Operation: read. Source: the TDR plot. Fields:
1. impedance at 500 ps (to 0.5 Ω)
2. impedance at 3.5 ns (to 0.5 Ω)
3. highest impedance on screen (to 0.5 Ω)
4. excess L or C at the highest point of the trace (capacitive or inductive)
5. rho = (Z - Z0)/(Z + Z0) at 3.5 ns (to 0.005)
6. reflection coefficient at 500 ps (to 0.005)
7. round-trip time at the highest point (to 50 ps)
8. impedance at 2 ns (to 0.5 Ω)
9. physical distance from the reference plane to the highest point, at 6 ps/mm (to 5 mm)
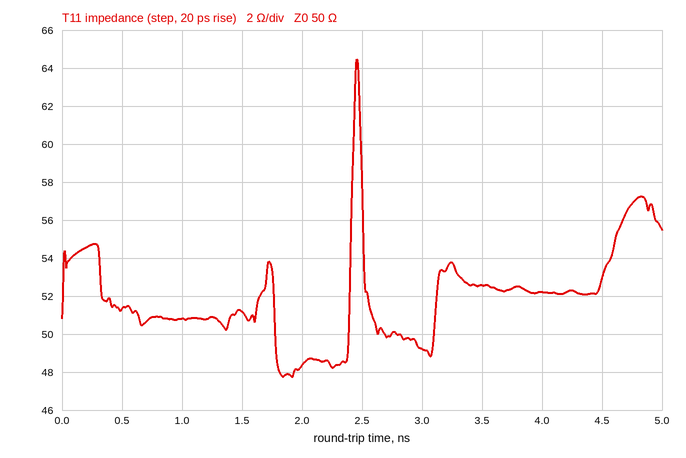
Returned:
51.5 Ω
52.5 Ω
64.5 Ω
inductive
+0.025
+0.015
2.45 ns
48.5 Ω
205 mm
